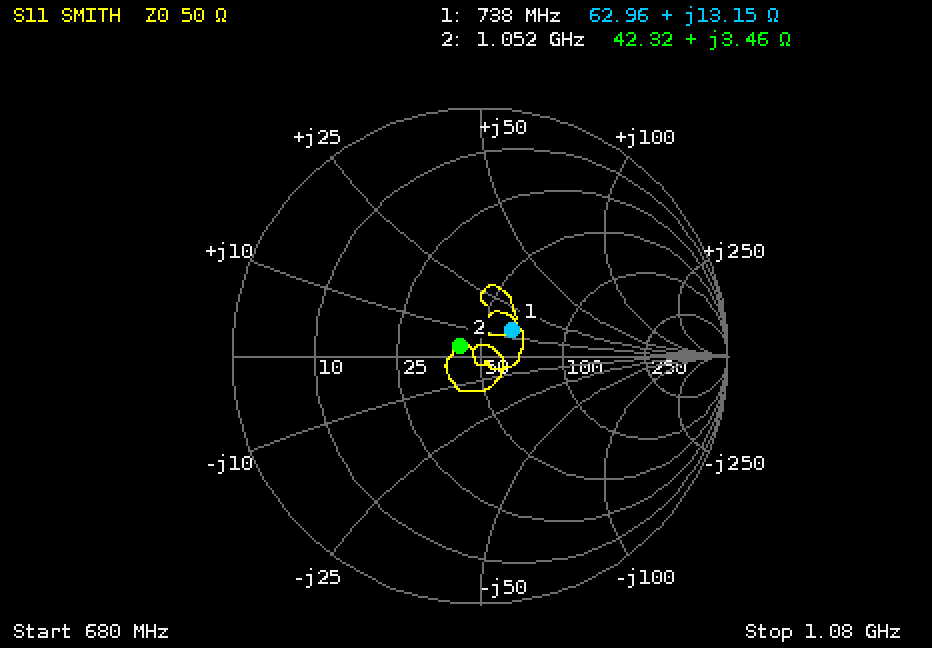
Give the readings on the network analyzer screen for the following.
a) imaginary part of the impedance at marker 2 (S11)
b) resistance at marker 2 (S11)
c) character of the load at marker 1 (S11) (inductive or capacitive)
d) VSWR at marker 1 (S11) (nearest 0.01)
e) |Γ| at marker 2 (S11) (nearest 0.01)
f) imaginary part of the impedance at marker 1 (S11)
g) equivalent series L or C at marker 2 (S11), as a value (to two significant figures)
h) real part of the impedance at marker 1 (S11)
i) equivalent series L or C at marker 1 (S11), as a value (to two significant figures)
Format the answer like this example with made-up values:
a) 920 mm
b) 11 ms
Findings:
a) +3.46 Ω
b) 42.32 Ω
c) inductive
d) 1.39
e) 0.09
f) +13.15 Ω
g) 520 pH
h) 62.96 Ω
i) 2.8 nH
